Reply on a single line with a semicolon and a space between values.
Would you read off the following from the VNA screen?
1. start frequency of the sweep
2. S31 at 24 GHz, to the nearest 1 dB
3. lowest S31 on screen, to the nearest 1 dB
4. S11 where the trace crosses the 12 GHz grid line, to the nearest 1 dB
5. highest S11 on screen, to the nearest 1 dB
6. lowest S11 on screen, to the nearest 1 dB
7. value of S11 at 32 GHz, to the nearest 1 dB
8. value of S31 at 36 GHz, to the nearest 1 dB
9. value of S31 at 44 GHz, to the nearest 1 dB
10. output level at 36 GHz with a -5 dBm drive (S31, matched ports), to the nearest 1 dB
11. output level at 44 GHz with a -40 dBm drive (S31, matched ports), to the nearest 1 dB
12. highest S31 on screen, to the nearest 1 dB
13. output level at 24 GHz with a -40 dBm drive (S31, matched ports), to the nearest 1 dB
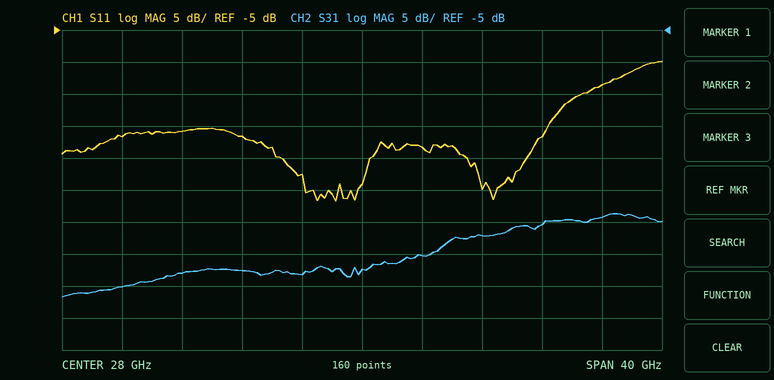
8 GHz; -43 dB; -47 dB; -22 dB; -10 dB; -32 dB; -23 dB; -37 dB; -34 dB; -42 dBm; -74 dBm; -34 dB; -83 dBm
